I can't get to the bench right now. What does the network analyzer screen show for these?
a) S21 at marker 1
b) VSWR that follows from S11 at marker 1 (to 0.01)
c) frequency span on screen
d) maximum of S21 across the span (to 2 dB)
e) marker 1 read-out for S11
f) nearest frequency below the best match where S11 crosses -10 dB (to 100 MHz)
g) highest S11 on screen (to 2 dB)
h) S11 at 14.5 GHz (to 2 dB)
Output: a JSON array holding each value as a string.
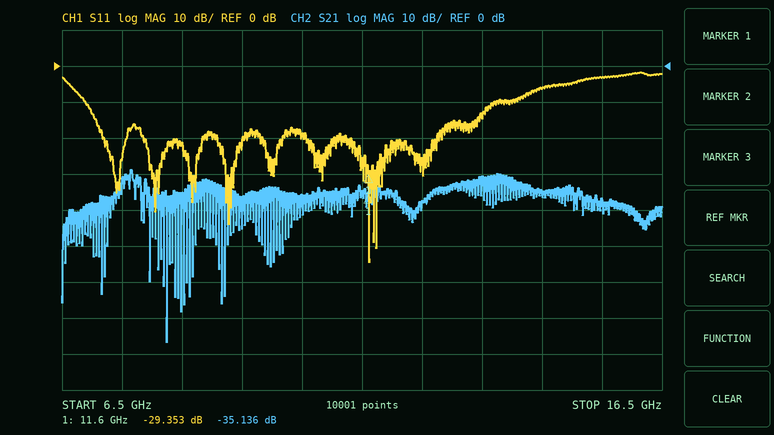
["-35.136 dB", "1.07", "10 GHz", "-28 dB", "-29.353 dB", "6.9 GHz", "-2 dB", "-6 dB"]
